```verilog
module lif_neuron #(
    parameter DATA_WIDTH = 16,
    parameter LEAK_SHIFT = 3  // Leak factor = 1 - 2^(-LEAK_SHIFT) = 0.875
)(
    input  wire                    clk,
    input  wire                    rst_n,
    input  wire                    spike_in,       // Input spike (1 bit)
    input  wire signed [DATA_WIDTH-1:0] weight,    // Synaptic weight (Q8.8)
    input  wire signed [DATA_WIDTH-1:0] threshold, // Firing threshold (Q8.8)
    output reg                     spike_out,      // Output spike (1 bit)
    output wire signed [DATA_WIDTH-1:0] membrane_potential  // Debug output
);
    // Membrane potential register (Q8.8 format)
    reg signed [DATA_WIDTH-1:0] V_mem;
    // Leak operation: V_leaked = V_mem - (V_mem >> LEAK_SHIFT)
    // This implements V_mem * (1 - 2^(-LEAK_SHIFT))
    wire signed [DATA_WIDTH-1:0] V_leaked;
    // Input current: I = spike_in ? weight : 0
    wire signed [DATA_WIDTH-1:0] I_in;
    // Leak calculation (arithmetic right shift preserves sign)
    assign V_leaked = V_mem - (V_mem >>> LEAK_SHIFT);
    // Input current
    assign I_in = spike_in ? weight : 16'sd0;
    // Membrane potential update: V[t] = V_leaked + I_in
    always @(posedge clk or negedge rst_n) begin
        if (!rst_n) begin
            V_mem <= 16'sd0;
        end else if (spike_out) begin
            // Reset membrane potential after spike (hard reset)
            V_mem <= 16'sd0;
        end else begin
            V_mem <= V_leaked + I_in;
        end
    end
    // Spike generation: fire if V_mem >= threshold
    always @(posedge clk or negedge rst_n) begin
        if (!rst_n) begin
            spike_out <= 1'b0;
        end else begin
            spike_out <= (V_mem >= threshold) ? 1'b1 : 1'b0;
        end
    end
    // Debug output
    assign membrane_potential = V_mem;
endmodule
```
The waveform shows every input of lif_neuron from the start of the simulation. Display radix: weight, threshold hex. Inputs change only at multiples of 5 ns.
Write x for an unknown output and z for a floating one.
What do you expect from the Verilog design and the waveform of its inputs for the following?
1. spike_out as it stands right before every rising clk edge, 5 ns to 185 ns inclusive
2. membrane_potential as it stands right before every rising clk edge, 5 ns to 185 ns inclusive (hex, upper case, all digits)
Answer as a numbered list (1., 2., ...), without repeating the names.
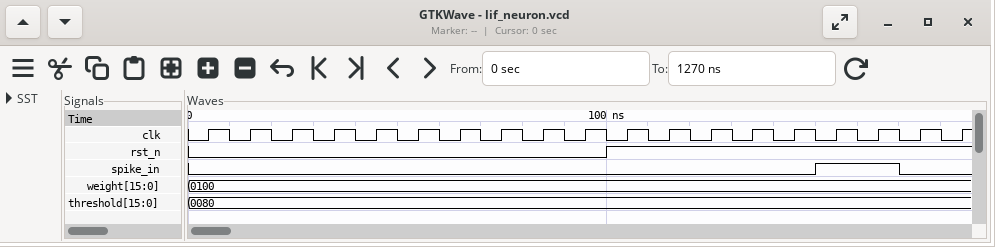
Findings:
1. 0 0 0 0 0 0 0 0 0 0 0 0 0 0 0 0 0 1 1
2. 0000, 0000, 0000, 0000, 0000, 0000, 0000, 0000, 0000, 0000, 0000, 0000, 0000, 0000, 0000, 0000, 0100, 01E0, 0000
